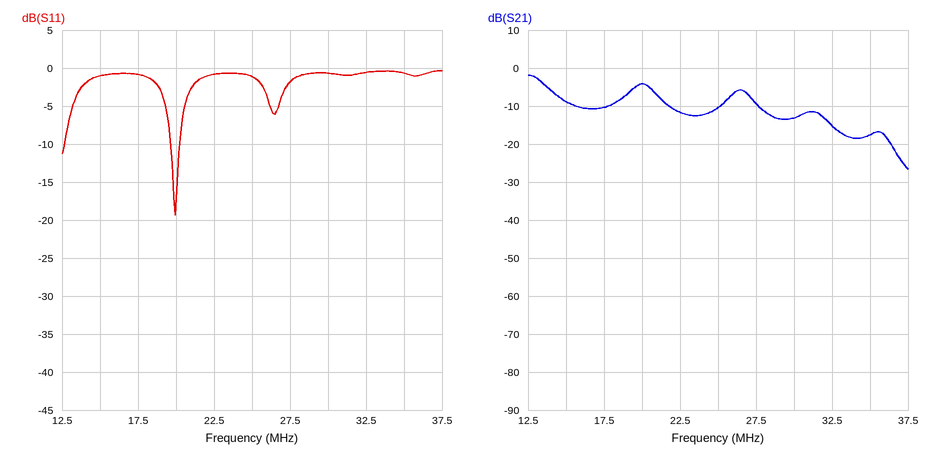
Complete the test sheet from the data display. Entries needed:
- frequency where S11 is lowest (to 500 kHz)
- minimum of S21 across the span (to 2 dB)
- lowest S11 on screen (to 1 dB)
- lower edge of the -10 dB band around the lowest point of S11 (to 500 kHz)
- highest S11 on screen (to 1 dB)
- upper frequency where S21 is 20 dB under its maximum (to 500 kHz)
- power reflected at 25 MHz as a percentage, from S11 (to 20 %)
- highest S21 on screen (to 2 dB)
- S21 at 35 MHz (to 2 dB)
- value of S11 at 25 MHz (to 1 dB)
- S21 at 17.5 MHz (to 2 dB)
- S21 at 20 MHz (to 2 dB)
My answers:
20.0 MHz
-26 dB
-19 dB
19.5 MHz
0 dB
36.5 MHz
80 %
-2 dB
-18 dB
-1 dB
-10 dB
-4 dB
